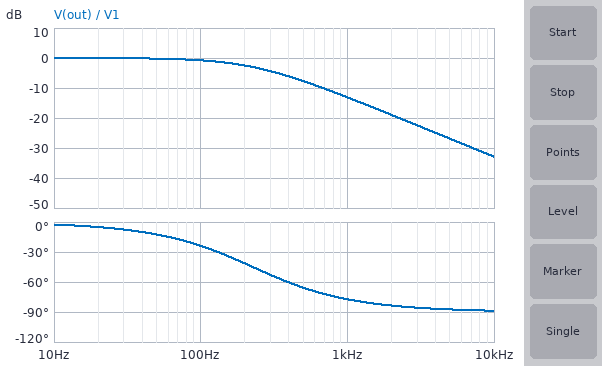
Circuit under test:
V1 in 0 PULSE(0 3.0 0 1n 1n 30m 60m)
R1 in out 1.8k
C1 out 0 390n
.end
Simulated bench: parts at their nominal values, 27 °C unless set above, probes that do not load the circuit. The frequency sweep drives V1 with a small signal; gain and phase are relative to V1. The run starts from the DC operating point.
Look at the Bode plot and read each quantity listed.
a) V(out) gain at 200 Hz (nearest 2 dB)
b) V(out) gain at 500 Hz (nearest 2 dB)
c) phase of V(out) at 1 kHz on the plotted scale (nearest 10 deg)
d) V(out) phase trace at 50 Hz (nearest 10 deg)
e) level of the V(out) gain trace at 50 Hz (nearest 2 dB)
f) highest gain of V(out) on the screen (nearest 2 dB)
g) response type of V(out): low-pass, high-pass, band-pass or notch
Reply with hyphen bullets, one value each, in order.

- -2 dB
- -8 dB
- -80 deg
- -10 deg
- 0 dB
- 0 dB
- low-pass
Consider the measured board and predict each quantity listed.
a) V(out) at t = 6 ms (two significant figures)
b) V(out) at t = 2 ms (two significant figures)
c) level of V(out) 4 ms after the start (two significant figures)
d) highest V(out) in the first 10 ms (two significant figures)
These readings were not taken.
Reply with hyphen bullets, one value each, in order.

- 3.0 V
- 2.8 V
- 3.0 V
- 3.0 V
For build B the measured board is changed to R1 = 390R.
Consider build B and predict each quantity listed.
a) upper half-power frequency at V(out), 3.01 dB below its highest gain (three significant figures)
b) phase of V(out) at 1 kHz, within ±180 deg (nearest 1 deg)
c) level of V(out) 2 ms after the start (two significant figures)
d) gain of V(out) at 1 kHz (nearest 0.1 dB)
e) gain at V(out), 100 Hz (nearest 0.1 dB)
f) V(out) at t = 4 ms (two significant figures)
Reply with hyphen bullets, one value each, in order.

- 1.05 kHz
- -44 deg
- 3.0 V
- -2.8 dB
- 0 dB
- 3.0 V
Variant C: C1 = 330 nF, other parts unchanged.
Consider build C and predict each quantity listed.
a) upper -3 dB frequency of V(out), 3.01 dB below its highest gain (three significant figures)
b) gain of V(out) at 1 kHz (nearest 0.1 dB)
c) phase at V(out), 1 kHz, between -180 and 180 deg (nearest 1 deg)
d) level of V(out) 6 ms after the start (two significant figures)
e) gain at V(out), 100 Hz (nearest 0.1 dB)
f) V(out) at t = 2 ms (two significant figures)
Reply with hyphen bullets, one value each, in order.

- 268 Hz
- -11.7 dB
- -75 deg
- 3.0 V
- -0.6 dB
- 2.9 V
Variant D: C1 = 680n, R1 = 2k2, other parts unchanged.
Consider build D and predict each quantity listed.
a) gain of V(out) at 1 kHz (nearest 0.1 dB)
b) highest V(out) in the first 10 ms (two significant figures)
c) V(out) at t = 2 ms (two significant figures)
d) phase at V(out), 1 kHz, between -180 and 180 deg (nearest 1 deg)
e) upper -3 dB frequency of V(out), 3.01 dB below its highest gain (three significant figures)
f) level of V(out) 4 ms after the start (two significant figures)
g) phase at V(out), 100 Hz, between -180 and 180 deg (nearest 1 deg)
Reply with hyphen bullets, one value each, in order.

- -19.5 dB
- 3.0 V
- 2.2 V
- -84 deg
- 106 Hz
- 2.8 V
- -43 deg
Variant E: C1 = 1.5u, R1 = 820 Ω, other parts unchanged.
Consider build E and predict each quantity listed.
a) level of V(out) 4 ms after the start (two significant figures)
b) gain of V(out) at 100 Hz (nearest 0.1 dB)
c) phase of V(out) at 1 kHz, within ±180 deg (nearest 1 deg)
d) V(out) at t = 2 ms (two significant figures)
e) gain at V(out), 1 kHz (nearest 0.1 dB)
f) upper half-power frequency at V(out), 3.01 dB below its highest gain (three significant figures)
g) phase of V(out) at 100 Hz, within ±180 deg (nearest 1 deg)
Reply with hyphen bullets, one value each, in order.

- 2.9 V
- -2.0 dB
- -83 deg
- 2.4 V
- -17.8 dB
- 129 Hz
- -38 deg
